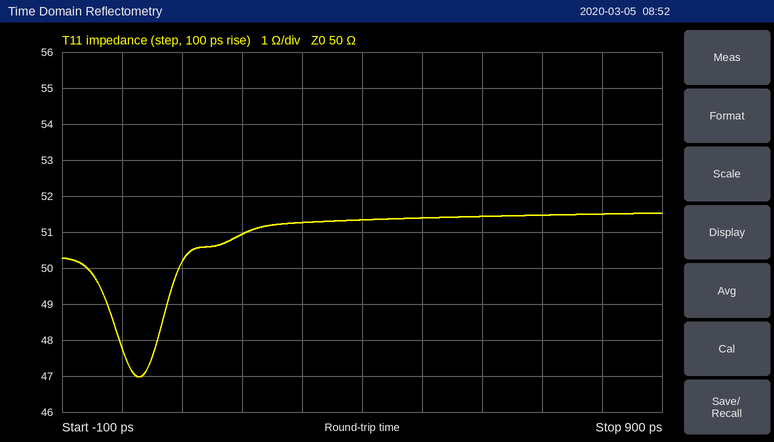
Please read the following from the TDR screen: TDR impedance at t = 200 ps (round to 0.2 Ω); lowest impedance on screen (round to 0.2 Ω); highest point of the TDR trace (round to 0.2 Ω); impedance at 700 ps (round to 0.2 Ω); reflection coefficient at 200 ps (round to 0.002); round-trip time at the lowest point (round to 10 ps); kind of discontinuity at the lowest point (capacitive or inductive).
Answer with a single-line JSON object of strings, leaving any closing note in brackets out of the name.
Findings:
{"TDR impedance at t = 200 ps": "51.0 Ω", "lowest impedance on screen": "47.0 Ω", "highest point of the TDR trace": "51.6 Ω", "impedance at 700 ps": "51.4 Ω", "reflection coefficient at 200 ps": "+0.010", "round-trip time at the lowest point": "30 ps", "kind of discontinuity at the lowest point": "capacitive"}
